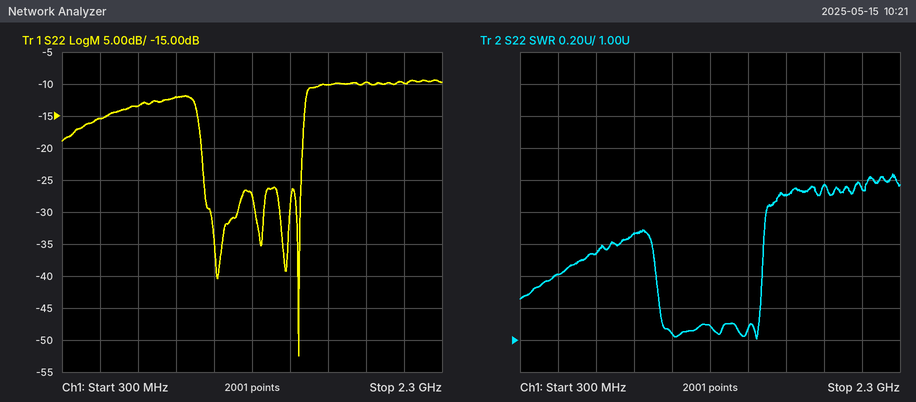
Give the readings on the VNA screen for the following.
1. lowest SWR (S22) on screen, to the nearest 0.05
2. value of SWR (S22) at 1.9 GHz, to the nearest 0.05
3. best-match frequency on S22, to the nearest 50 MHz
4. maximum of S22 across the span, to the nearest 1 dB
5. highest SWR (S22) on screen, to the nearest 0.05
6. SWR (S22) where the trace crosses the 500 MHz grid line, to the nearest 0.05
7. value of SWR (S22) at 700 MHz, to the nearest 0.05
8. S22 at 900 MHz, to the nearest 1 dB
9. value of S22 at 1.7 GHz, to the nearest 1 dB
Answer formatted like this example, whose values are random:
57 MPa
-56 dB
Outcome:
1.00
1.95
1.55 GHz
-9 dB
2.05
1.40
1.55
-12 dB
-10 dB
